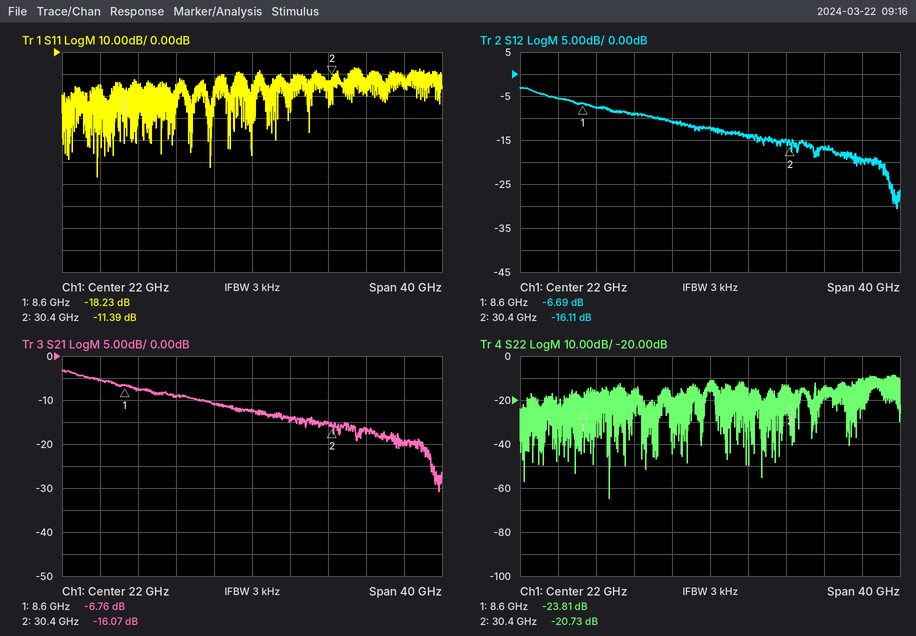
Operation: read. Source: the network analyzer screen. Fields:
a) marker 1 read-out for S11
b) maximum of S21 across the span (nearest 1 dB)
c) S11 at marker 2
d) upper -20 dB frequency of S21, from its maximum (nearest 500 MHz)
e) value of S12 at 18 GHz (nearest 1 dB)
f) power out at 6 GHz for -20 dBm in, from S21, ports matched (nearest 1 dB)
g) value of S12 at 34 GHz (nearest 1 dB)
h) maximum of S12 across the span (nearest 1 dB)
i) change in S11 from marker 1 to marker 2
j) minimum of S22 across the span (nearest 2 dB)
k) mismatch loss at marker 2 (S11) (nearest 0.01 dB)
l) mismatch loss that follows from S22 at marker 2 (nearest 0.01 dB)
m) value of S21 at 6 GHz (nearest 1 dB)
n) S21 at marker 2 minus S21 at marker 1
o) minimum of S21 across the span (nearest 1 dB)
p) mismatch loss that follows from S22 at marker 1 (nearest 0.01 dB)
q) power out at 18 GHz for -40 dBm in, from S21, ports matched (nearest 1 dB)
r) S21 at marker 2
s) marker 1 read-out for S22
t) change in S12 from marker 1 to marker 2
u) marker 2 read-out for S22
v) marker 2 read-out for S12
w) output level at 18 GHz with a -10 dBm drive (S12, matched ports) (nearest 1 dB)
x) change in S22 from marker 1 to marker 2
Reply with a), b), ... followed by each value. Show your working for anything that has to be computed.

a) -18.23 dB
b) -3 dB
c) -11.39 dB
d) 40.5 GHz
e) -11 dB
f) -20 dBm + (-5 dB) = -25 dBm
g) -17 dB
h) -3 dB
i) -11.39 − (-18.23) = 6.84 dB
j) -64 dB
k) −10 log10(1 − 10^(-11.39/10)) ≈ 0.33 dB
l) −10 log10(1 − 10^(-20.73/10)) ≈ 0.04 dB
m) -5 dB
n) -16.07 − (-6.76) = -9.31 dB
o) -31 dB
p) −10 log10(1 − 10^(-23.81/10)) ≈ 0.02 dB
q) -40 dBm + (-11 dB) = -51 dBm
r) -16.07 dB
s) -23.81 dB
t) -16.11 − (-6.69) = -9.42 dB
u) -20.73 dB
v) -16.11 dB
w) -10 dBm + (-11 dB) = -21 dBm
x) -20.73 − (-23.81) = 3.08 dB
